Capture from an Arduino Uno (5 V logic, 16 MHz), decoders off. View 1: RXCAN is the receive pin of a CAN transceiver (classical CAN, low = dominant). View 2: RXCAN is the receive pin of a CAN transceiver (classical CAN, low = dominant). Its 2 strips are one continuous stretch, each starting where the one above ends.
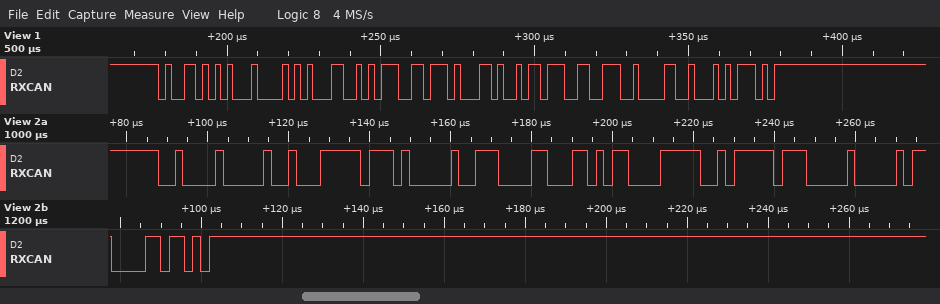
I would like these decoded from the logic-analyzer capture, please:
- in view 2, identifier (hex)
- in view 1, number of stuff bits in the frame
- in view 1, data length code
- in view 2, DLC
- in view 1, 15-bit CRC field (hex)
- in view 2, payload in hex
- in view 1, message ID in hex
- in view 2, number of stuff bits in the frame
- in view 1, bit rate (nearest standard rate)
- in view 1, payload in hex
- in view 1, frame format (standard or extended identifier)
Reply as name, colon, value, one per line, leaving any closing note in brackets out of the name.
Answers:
in view 2, identifier: 0x210
in view 1, number of stuff bits in the frame: 0
in view 1, data length code: 8
in view 2, DLC: 8
in view 1, 15-bit CRC field: 0x48AE
in view 2, payload in hex: FF 40 70 C6 B0 FA FF 00
in view 1, message ID in hex: 0x4D5
in view 2, number of stuff bits in the frame: 7
in view 1, bit rate: 500 kbit/s
in view 1, payload in hex: 54 65 73 74 69 6E 67 21
in view 1, frame format: standard
